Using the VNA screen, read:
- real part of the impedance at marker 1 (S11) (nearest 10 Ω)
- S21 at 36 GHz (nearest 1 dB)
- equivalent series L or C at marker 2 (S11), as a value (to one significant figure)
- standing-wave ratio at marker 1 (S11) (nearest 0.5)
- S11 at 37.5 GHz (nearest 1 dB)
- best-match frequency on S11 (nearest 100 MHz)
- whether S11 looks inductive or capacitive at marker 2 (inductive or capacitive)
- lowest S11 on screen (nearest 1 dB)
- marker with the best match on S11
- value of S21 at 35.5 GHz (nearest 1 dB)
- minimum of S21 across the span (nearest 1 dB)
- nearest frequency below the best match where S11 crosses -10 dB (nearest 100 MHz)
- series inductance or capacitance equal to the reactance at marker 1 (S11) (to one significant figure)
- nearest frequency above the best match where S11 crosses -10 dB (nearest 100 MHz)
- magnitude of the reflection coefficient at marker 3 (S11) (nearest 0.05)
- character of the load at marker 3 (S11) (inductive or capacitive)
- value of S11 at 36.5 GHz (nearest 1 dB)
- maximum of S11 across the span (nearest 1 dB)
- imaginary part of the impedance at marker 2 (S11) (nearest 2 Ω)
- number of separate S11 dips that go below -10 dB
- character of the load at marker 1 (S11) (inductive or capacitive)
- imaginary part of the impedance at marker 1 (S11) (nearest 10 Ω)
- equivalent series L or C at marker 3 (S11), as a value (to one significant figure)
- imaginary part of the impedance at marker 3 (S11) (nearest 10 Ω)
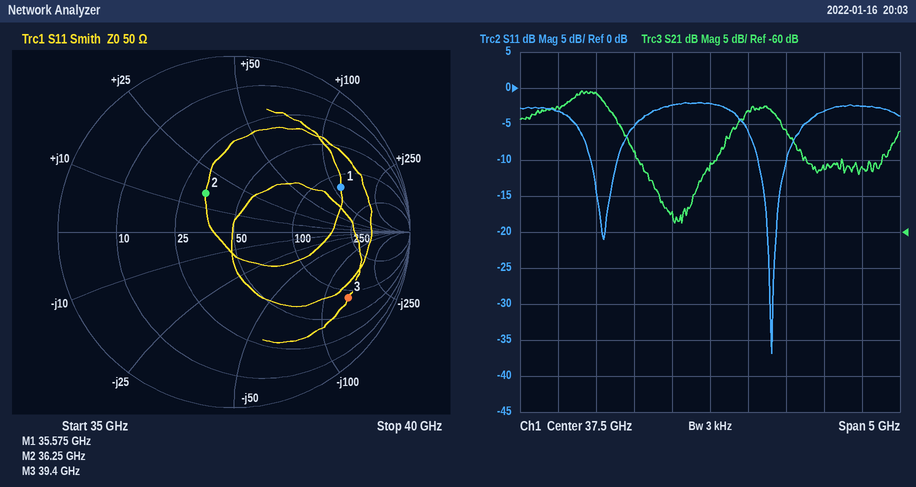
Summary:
130 Ω
-41 dB
70 pH
5.0
-2 dB
38.3 GHz
inductive
-37 dB
marker 2
-43 dB
-59 dB
38.1 GHz
500 pH
38.5 GHz
0.75
capacitive
-5 dB
-2 dB
+16 Ω
2
inductive
+120 Ω
30 fF
-140 Ω
